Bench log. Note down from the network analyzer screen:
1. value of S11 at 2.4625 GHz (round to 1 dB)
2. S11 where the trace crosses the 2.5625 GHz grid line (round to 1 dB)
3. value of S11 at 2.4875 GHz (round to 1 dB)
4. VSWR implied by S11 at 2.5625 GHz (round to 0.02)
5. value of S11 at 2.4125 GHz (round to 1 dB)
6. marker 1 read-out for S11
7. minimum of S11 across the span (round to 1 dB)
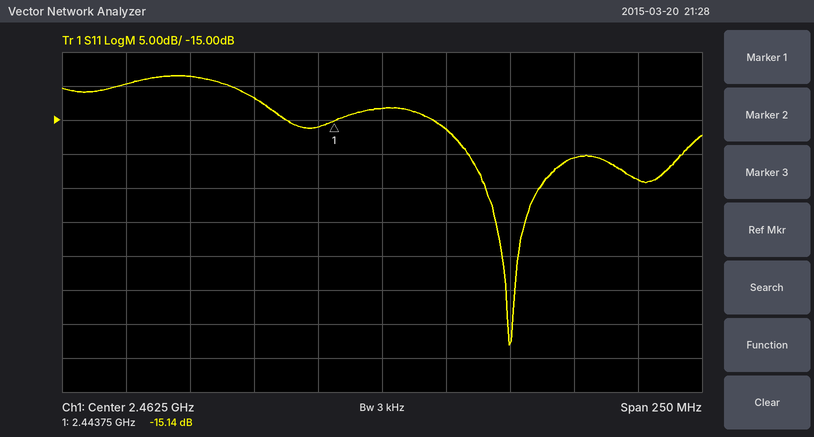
-13 dB
-24 dB
-16 dB
1.14
-12 dB
-15.14 dB
-48 dB
